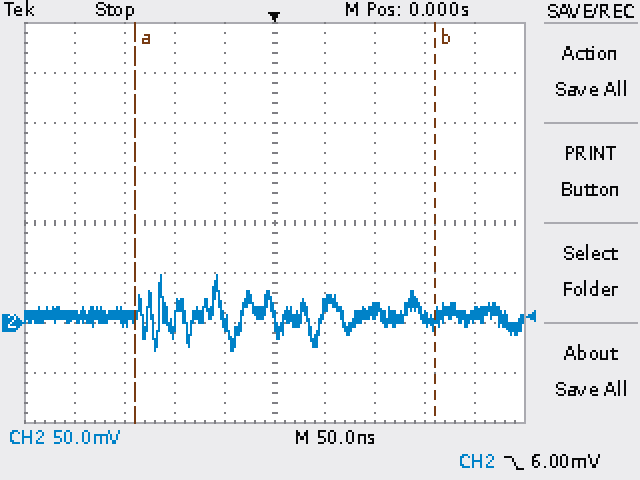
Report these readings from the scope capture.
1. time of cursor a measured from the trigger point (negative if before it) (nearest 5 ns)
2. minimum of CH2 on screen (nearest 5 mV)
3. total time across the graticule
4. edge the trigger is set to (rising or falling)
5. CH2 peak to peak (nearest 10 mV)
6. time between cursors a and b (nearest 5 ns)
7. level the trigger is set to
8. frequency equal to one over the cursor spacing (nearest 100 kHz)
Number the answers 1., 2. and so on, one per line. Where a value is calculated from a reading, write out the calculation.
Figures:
1. -140 ns
2. -30 mV
3. 500 ns
4. falling
5. 80 mV
6. 300 ns
7. 6.00 mV
8. 1 / 300 ns ≈ 3.3 MHz
